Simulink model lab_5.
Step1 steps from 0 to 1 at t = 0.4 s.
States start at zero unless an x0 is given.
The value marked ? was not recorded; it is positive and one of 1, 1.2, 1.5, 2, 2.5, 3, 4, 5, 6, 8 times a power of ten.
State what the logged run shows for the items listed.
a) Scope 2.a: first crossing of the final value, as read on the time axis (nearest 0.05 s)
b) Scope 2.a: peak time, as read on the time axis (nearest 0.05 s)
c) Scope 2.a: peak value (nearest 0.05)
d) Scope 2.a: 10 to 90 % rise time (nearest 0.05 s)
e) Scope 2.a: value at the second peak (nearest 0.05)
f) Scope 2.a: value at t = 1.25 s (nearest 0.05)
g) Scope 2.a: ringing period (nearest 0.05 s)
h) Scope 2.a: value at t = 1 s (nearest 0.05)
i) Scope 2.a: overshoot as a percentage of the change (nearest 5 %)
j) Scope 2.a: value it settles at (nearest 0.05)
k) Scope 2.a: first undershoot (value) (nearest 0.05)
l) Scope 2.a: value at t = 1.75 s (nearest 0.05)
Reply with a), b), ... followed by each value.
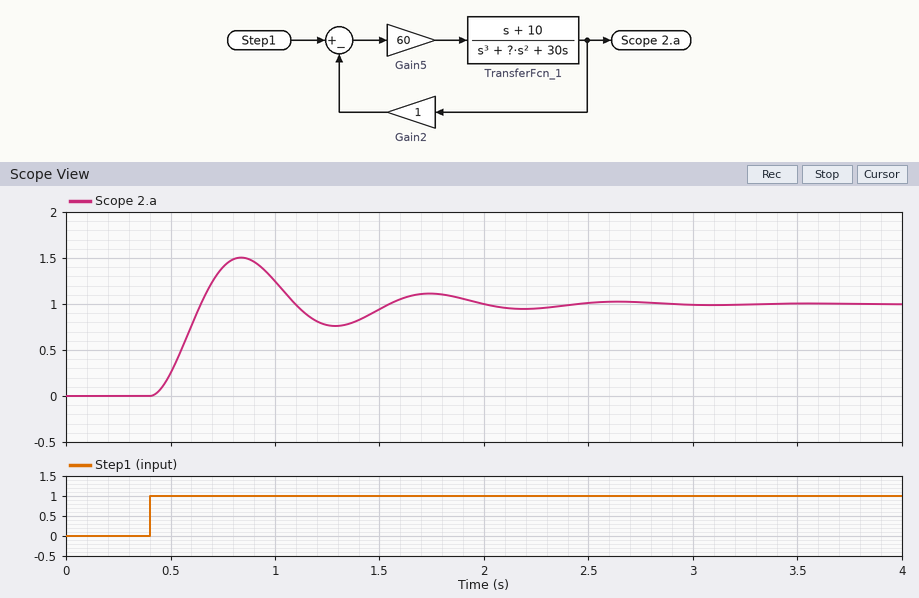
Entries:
a) 0.65 s
b) 0.85 s
c) 1.50
d) 0.15 s
e) 1.10
f) 0.75
g) 0.90 s
h) 1.25
i) 50 %
j) 1.00
k) 0.75
l) 1.10
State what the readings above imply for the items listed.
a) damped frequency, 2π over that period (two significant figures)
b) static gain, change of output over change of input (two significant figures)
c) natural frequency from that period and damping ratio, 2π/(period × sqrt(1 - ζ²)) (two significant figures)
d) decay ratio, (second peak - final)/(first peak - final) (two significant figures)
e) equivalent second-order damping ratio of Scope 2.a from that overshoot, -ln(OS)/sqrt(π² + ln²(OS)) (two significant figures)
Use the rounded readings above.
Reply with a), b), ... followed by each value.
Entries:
a) 7.0 rad/s
b) 1.0
c) 7.2 rad/s
d) 0.20
e) 0.22
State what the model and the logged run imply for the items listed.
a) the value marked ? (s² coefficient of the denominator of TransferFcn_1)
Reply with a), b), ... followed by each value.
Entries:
a) 15
